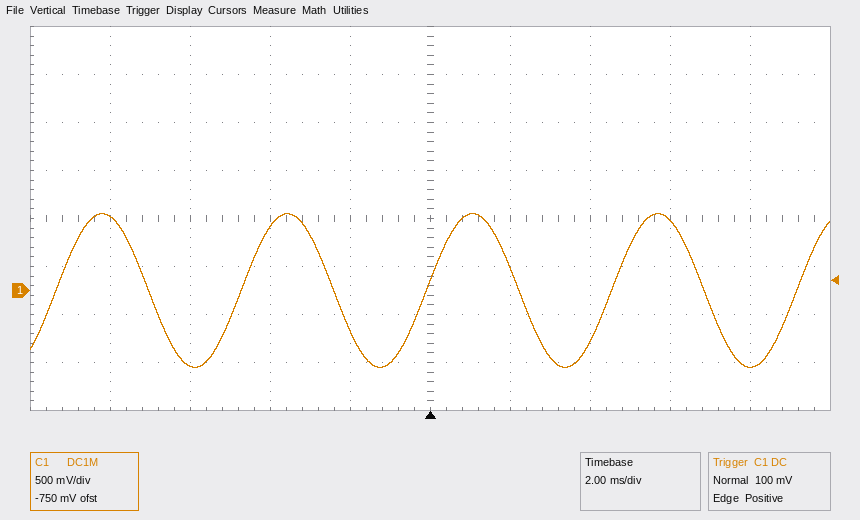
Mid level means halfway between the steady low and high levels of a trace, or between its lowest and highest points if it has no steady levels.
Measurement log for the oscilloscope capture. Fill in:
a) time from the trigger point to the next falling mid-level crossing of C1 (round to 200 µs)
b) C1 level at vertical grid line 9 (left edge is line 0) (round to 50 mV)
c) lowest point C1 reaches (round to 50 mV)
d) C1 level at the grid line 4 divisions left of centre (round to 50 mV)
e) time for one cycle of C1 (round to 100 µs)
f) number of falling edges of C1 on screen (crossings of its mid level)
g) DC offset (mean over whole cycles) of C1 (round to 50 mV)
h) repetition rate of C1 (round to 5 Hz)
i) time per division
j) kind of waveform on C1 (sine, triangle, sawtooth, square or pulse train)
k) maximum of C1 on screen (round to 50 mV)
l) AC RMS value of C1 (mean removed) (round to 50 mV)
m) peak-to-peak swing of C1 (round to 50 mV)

2.2 ms
-800 mV
-800 mV
750 mV
4.6 ms
4
0 mV
215 Hz
2 ms
sine
800 mV
550 mV
1.60 V
